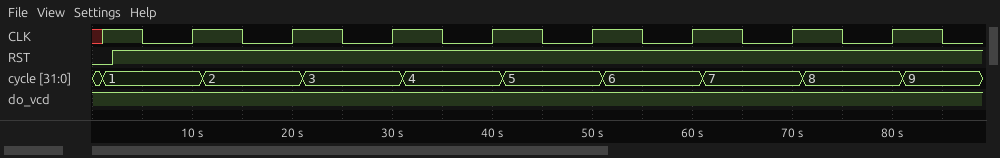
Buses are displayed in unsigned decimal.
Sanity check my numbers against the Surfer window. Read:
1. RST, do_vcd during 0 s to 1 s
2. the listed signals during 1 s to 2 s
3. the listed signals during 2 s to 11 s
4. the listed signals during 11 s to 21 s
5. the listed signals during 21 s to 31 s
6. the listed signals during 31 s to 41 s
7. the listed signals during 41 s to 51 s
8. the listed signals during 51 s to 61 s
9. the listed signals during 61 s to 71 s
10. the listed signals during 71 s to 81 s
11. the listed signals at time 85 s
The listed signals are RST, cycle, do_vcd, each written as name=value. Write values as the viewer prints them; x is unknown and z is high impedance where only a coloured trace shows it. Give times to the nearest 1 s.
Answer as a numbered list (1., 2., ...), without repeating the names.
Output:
1. RST=0, do_vcd=1
2. RST=0, cycle=1, do_vcd=1
3. RST=1, cycle=1, do_vcd=1
4. RST=1, cycle=2, do_vcd=1
5. RST=1, cycle=3, do_vcd=1
6. RST=1, cycle=4, do_vcd=1
7. RST=1, cycle=5, do_vcd=1
8. RST=1, cycle=6, do_vcd=1
9. RST=1, cycle=7, do_vcd=1
10. RST=1, cycle=8, do_vcd=1
11. RST=1, cycle=9, do_vcd=1
